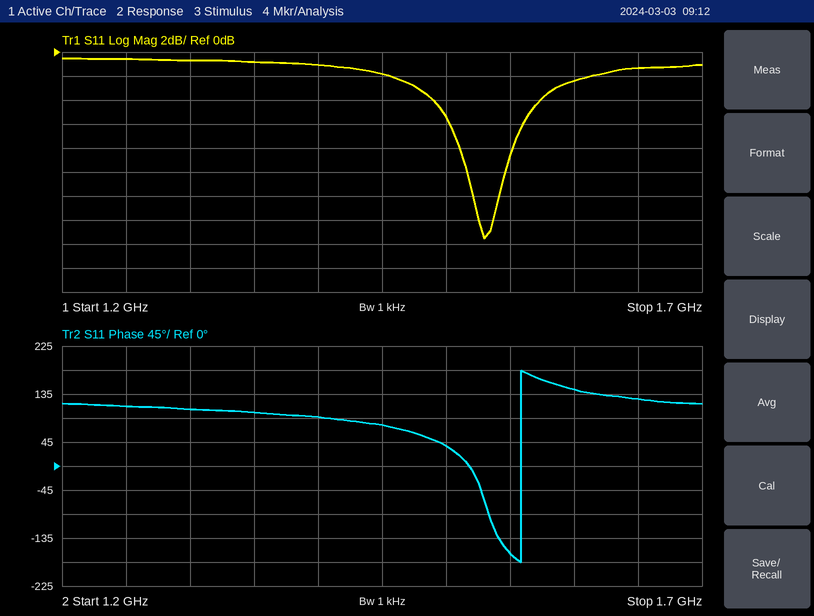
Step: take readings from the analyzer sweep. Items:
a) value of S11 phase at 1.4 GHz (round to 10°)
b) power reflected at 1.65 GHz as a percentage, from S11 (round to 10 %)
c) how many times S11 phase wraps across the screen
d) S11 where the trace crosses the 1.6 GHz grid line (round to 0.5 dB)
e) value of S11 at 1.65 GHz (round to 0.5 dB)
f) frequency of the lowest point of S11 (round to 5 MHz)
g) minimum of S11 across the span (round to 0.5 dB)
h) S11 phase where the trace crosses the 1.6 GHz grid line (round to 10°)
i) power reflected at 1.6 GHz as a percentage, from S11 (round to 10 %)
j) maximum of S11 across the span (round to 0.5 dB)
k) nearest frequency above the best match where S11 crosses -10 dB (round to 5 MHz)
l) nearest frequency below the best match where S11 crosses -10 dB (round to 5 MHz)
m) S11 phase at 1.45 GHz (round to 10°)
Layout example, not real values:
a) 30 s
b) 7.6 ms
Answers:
a) 90°
b) 70 %
c) 1
d) -2.5 dB
e) -1.5 dB
f) 1.530 GHz
g) -15.5 dB
h) 140°
i) 60 %
j) -0.5 dB
k) 1.545 GHz
l) 1.515 GHz
m) 80°
